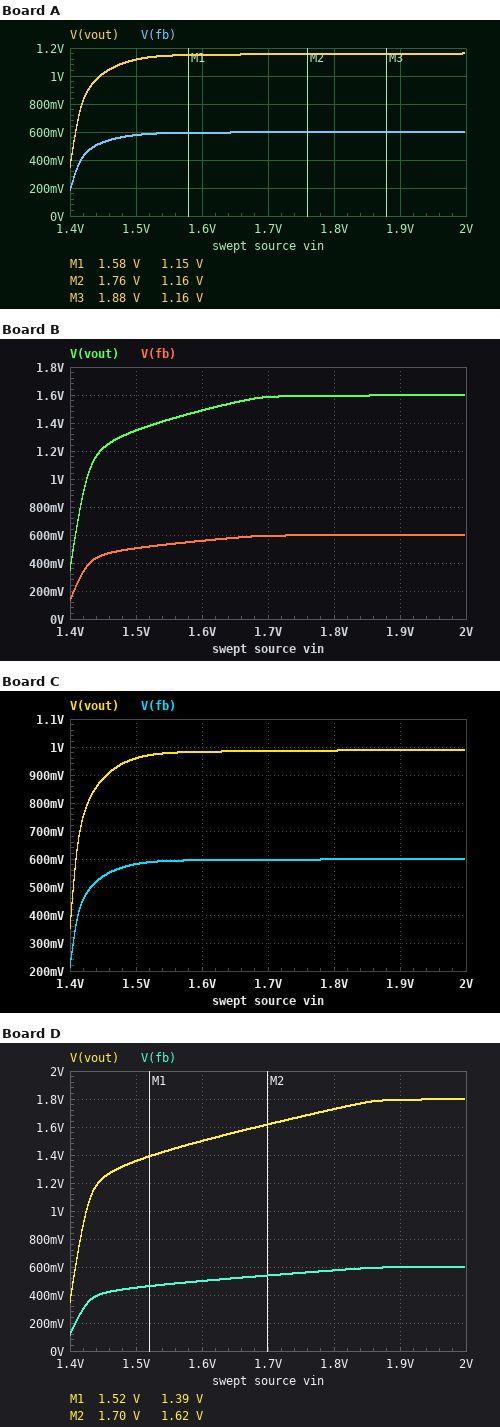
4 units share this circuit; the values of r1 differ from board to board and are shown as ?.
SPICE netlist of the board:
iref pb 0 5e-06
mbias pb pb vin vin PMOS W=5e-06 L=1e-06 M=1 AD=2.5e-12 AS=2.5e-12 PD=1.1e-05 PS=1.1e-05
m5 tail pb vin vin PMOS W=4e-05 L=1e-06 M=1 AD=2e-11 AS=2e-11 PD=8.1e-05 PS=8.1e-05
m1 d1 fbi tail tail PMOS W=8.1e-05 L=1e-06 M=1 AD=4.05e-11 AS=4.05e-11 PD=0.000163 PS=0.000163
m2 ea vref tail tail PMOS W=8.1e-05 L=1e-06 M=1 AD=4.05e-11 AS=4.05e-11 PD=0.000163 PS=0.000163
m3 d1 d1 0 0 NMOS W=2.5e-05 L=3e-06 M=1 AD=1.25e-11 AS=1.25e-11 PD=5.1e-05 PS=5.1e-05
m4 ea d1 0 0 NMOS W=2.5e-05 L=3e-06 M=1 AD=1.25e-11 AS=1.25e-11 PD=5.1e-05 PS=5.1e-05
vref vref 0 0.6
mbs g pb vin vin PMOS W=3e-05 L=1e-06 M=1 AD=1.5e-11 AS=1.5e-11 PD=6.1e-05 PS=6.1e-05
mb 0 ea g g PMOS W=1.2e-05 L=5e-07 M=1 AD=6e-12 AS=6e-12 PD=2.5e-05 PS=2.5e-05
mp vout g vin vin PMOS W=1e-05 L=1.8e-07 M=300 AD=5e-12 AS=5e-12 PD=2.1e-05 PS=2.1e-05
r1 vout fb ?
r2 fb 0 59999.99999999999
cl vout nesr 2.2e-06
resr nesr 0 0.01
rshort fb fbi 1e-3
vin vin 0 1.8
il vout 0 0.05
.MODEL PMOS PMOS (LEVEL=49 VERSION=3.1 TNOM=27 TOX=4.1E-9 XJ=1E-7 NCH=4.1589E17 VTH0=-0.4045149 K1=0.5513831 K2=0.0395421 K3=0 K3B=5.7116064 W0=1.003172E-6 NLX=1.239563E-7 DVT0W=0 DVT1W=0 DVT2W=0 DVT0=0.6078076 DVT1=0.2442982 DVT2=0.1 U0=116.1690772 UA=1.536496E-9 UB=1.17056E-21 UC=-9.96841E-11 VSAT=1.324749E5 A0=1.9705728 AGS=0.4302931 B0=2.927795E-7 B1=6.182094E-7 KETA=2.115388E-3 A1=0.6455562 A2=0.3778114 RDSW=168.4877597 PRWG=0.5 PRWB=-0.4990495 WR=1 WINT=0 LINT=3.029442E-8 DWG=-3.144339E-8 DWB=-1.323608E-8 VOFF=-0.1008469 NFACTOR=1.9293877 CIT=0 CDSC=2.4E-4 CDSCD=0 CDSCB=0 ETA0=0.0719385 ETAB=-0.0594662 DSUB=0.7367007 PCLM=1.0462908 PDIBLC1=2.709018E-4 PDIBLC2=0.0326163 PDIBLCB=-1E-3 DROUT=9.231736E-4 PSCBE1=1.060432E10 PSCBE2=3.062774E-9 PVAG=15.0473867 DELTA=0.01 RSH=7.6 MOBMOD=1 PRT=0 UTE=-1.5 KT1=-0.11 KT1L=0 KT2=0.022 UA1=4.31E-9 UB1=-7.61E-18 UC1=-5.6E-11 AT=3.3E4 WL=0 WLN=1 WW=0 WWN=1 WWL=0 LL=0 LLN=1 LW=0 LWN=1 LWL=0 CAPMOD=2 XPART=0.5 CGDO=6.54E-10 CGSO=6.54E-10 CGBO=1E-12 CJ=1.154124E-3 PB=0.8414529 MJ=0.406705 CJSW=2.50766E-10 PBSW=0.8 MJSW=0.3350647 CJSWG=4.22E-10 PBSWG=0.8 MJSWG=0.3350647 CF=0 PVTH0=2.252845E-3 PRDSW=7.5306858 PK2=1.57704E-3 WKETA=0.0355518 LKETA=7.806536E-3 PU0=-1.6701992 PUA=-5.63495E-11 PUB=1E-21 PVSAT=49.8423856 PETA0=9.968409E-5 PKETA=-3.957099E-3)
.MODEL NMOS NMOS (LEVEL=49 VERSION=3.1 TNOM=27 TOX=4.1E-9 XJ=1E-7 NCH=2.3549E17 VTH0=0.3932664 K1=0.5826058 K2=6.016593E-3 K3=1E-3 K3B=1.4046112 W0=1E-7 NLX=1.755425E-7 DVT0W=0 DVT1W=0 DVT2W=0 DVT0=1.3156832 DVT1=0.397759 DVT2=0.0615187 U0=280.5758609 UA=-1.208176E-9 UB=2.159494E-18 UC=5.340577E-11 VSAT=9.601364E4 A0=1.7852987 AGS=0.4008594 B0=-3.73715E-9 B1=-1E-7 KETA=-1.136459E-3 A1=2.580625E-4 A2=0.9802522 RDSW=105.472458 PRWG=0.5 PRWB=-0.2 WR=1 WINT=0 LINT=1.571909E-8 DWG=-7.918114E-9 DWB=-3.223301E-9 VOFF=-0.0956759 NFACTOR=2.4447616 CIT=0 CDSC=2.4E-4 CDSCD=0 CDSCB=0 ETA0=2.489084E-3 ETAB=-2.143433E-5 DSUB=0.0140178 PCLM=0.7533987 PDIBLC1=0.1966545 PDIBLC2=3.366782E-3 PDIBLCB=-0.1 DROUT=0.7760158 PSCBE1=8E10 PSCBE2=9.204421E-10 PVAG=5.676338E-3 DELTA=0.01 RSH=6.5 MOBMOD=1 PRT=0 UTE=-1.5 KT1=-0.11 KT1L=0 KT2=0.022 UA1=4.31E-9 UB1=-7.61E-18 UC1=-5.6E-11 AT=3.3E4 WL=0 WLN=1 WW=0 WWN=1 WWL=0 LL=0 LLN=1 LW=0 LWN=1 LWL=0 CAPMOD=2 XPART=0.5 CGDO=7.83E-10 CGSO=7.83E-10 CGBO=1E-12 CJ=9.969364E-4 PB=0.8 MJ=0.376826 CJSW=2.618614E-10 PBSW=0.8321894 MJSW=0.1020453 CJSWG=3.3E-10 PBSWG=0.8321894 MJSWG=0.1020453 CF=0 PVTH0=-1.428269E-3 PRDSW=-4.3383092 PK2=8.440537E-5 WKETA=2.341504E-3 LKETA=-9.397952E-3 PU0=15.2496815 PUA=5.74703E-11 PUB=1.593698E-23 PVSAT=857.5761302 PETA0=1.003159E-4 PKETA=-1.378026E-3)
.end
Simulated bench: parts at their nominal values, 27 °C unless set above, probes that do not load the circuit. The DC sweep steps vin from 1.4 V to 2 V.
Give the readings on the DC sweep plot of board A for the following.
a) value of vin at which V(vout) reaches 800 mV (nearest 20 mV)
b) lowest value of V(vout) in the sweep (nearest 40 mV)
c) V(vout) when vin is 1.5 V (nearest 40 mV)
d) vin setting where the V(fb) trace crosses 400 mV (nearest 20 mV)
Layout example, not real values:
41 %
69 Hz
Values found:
1.42 V
360 mV
1.12 V
1.42 V
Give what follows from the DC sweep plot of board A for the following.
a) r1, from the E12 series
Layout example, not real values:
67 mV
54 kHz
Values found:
56 kΩ
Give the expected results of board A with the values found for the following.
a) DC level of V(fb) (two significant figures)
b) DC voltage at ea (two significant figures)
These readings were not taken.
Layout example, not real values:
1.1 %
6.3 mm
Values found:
600 mV
390 mV
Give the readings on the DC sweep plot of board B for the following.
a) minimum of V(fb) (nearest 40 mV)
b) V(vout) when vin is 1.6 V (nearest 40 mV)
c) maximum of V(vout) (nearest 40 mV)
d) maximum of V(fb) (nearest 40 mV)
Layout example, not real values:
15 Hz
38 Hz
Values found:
120 mV
1.48 V
1.60 V
600 mV
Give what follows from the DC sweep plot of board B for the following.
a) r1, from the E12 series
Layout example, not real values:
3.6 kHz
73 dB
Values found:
100 kΩ
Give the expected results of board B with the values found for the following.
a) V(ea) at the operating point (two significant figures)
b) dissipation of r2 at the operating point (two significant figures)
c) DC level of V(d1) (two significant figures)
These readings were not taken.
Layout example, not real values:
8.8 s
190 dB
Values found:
350 mV
6.0 µW
560 mV
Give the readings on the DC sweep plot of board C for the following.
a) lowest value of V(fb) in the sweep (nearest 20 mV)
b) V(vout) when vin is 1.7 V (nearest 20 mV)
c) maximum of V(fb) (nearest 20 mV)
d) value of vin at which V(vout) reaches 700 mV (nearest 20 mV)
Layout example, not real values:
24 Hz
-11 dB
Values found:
220 mV
980 mV
600 mV
1.42 V
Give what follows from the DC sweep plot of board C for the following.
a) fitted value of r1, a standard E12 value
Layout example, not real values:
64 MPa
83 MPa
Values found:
39 kΩ
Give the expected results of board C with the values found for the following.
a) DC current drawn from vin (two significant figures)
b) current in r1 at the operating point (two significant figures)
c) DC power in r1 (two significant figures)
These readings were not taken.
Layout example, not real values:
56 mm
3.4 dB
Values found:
50 mA
10 µA
3.9 µW
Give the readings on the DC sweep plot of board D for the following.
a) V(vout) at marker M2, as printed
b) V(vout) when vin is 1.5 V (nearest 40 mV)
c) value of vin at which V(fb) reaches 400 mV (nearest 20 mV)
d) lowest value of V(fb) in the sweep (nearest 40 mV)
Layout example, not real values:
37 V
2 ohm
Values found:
1.62 V
1.36 V
1.44 V
120 mV
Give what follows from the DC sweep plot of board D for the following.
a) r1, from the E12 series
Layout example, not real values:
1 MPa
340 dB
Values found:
120 kΩ
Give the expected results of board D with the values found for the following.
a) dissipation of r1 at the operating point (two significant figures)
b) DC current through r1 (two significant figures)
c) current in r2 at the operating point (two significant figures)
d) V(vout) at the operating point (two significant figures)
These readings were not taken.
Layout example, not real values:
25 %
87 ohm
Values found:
11 µW
9.6 µA
9.6 µA
1.7 V
